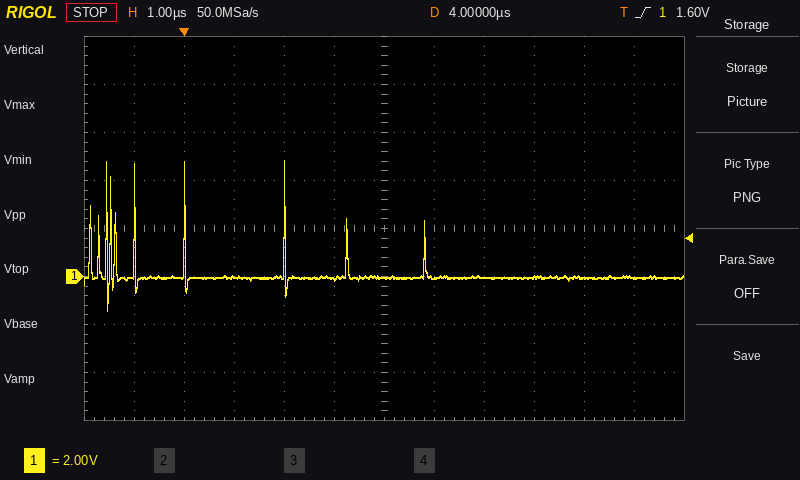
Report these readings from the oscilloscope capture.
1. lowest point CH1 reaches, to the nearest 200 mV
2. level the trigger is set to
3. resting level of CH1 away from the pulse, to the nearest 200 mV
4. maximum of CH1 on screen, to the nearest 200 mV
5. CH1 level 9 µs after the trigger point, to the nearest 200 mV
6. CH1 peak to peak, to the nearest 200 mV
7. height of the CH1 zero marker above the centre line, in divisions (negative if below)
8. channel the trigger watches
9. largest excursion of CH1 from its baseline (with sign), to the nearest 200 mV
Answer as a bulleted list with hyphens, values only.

- -1.4 V
- 1.60 V
- 0.0 V
- 4.8 V
- 0.0 V
- 6.2 V
- -1.0 div
- CH1
- +4.8 V
